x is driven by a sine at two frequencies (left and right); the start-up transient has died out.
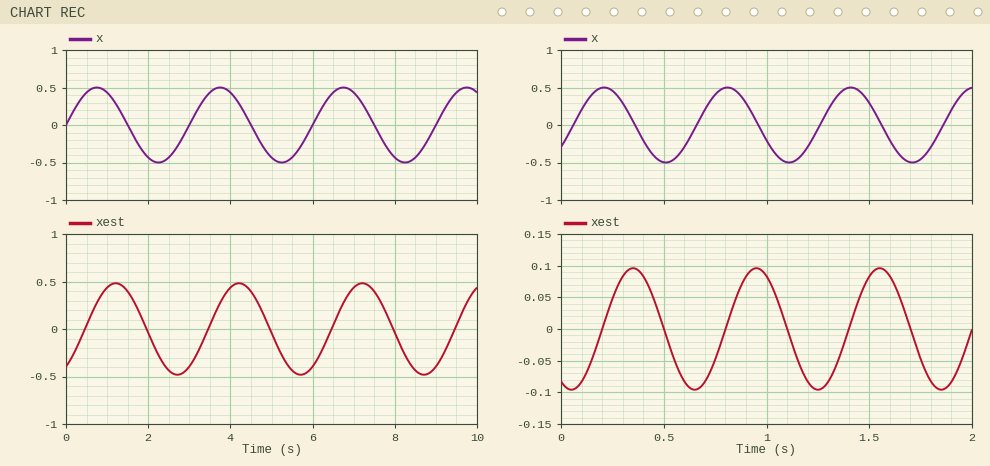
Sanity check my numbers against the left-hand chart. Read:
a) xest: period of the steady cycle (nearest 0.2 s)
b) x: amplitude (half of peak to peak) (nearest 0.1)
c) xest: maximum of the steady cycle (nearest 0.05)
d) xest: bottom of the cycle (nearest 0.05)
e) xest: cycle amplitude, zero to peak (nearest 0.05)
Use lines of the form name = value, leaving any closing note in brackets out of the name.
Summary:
xest: period of the steady cycle = 3.0 s
x: amplitude (half of peak to peak) = 0.5
xest: maximum of the steady cycle = 0.50
xest: bottom of the cycle = -0.50
xest: cycle amplitude, zero to peak = 0.50
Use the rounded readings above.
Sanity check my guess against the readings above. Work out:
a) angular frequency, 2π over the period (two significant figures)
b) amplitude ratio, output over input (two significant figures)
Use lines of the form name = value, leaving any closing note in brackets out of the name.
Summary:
angular frequency, 2π over the period = 2.1 rad/s
amplitude ratio, output over input = 1.0
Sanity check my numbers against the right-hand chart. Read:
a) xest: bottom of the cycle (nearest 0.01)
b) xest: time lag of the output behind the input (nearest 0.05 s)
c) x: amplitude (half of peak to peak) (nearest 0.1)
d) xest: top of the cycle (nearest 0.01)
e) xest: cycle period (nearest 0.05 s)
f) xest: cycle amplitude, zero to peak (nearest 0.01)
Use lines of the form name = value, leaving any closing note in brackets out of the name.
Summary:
xest: bottom of the cycle = -0.10
xest: time lag of the output behind the input = 0.15 s
x: amplitude (half of peak to peak) = 0.5
xest: top of the cycle = 0.10
xest: cycle period = 0.60 s
xest: cycle amplitude, zero to peak = 0.10
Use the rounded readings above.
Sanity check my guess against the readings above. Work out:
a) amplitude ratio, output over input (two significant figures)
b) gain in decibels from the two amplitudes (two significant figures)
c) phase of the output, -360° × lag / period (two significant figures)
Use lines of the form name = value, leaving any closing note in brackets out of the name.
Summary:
amplitude ratio, output over input = 0.20
gain in decibels from the two amplitudes = -14 dB
phase of the output, -360° × lag / period = -90°
